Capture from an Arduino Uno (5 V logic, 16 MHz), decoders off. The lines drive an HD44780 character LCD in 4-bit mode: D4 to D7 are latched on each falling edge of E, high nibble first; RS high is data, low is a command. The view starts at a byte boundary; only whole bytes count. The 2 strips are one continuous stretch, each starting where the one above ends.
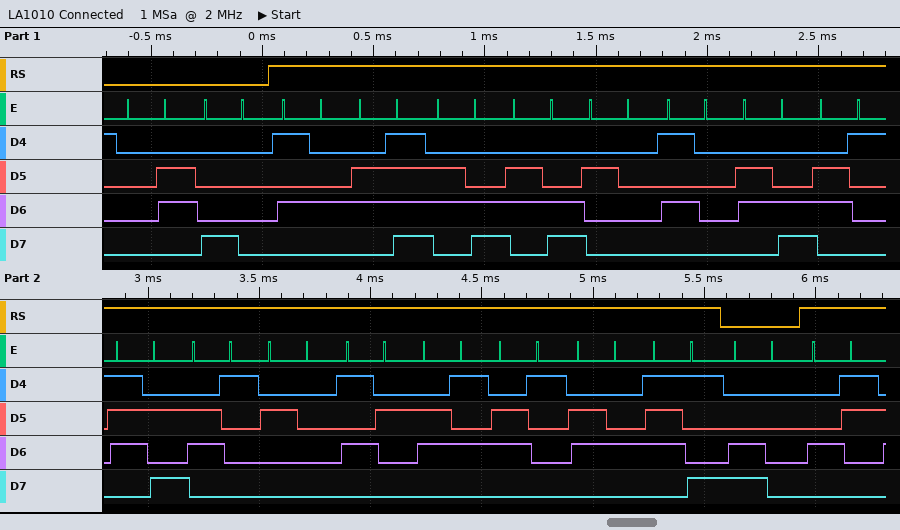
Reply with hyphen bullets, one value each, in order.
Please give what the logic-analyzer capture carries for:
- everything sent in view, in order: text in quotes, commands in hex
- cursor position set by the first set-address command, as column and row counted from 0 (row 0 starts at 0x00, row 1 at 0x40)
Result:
- 0x06 0x80 "Toll Plaza Ready" 0xC0 "C"
- column 0, row 0
